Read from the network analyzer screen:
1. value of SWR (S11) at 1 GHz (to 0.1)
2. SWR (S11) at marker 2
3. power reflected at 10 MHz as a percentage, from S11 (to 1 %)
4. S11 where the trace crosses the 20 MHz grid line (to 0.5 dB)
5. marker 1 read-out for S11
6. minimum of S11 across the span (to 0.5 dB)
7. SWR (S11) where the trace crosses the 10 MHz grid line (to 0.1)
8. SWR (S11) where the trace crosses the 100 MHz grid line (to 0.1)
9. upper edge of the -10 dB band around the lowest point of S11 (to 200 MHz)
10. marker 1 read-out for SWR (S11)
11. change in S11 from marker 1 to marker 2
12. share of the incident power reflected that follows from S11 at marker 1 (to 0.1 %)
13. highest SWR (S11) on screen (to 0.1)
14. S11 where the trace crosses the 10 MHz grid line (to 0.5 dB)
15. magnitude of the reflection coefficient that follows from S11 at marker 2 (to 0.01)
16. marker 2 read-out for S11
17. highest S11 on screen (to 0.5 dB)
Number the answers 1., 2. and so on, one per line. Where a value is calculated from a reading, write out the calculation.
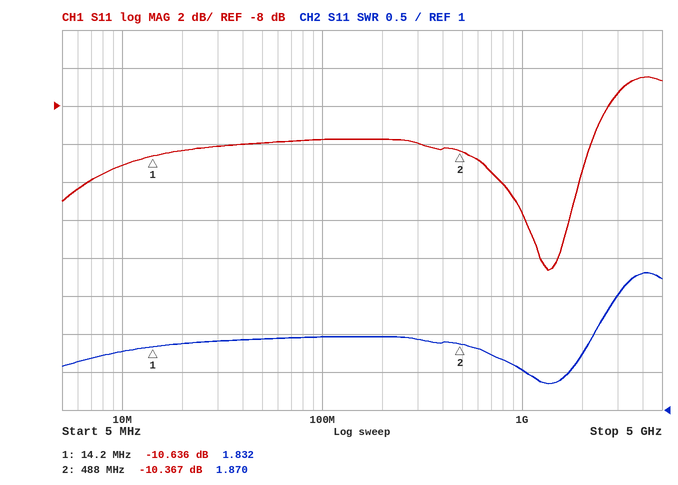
1. 1.5
2. 1.870
3. 10^(-11/10) ≈ 8 %
4. -10.5 dB
5. -10.636 dB
6. -16.5 dB
7. 1.8
8. 2.0
9. 2.2 GHz
10. 1.832
11. -10.367 − (-10.636) = 0.269 dB
12. 10^(-10.636/10) ≈ 8.6 %
13. 2.8
14. -11.0 dB
15. 10^(-10.367/20) ≈ 0.30
16. -10.367 dB
17. -6.5 dB
